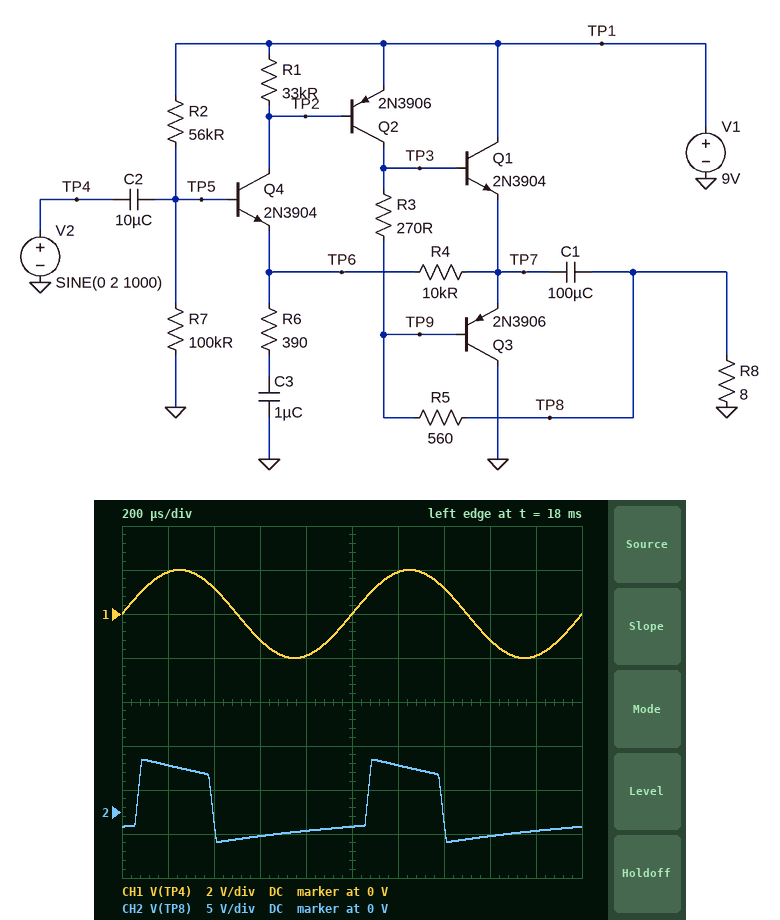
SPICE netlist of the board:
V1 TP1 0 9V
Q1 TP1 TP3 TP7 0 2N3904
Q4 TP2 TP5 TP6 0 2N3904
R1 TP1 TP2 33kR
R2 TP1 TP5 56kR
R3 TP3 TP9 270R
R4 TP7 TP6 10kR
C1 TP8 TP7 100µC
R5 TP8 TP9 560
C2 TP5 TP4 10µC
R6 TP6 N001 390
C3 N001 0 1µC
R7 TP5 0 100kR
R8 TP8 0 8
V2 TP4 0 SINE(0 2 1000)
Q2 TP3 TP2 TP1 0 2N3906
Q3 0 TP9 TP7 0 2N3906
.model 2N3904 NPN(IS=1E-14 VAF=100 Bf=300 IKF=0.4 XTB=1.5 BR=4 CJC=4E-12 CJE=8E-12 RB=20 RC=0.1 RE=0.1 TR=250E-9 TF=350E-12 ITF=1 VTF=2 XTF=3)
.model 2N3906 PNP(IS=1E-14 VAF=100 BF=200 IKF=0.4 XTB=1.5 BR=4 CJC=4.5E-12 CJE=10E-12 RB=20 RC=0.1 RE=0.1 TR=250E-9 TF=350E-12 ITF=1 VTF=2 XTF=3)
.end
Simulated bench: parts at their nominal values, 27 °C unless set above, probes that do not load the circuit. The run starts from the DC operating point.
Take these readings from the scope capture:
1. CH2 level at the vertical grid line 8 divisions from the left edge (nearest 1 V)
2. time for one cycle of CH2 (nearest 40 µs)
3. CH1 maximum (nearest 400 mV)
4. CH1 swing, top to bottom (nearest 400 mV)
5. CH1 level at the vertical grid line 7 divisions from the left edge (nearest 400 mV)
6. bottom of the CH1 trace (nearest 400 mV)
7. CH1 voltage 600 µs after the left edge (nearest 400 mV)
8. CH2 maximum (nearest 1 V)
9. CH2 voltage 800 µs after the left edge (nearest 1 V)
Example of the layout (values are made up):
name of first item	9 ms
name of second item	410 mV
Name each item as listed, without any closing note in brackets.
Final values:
CH2 level at the vertical grid line 8 divisions from the left edge	-3 V
time for one cycle of CH2	1.00 ms
CH1 maximum	2.0 V
CH1 swing, top to bottom	4.0 V
CH1 level at the vertical grid line 7 divisions from the left edge	1.2 V
bottom of the CH1 trace	-2.0 V
CH1 voltage 600 µs after the left edge	-1.2 V
CH2 maximum	6 V
CH2 voltage 800 µs after the left edge	-2 V
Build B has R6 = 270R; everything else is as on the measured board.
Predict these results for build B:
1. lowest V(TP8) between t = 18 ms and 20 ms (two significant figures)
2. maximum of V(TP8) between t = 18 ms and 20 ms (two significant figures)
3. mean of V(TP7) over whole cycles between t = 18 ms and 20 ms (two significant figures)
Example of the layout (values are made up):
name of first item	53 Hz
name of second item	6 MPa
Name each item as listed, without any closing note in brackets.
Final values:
lowest V(TP8) between t = 18 ms and 20 ms	-3.2 V
maximum of V(TP8) between t = 18 ms and 20 ms	6.1 V
mean of V(TP7) over whole cycles between t = 18 ms and 20 ms	2.5 V
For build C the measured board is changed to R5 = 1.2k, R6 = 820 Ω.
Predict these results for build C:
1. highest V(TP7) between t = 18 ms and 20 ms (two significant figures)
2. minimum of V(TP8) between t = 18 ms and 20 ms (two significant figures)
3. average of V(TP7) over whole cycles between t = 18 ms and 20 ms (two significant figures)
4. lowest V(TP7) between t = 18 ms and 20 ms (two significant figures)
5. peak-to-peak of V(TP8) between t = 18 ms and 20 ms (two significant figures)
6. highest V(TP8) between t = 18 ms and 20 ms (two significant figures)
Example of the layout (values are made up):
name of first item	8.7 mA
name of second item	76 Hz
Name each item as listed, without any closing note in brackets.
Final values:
highest V(TP7) between t = 18 ms and 20 ms	8.0 V
minimum of V(TP8) between t = 18 ms and 20 ms	-2.7 V
average of V(TP7) over whole cycles between t = 18 ms and 20 ms	3.8 V
lowest V(TP7) between t = 18 ms and 20 ms	1.2 V
peak-to-peak of V(TP8) between t = 18 ms and 20 ms	7.5 V
highest V(TP8) between t = 18 ms and 20 ms	4.8 V
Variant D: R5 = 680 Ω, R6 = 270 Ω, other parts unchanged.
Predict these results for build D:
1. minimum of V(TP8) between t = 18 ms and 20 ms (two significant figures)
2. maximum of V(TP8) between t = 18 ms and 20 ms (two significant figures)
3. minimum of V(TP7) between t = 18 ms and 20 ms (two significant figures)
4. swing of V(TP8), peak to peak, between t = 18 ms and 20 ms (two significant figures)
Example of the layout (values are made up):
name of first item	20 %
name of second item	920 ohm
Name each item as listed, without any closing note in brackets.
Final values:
minimum of V(TP8) between t = 18 ms and 20 ms	-3.1 V
maximum of V(TP8) between t = 18 ms and 20 ms	6.1 V
minimum of V(TP7) between t = 18 ms and 20 ms	280 mV
swing of V(TP8), peak to peak, between t = 18 ms and 20 ms	9.1 V
